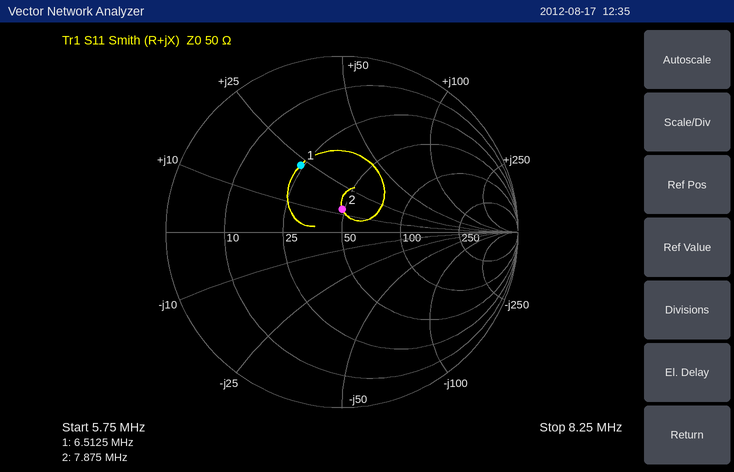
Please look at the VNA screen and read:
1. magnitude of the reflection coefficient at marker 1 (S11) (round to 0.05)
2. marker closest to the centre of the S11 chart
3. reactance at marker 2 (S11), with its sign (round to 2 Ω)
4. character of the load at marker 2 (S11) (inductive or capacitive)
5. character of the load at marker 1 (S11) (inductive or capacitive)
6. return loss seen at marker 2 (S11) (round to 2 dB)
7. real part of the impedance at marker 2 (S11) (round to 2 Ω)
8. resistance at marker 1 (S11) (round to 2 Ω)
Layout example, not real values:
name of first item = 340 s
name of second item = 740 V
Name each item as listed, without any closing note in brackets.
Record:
magnitude of the reflection coefficient at marker 1 (S11) = 0.45
marker closest to the centre of the S11 chart = marker 2
reactance at marker 2 (S11), with its sign = +12 Ω
character of the load at marker 2 (S11) = inductive
character of the load at marker 1 (S11) = inductive
return loss seen at marker 2 (S11) = 18 dB
real part of the impedance at marker 2 (S11) = 48 Ω
resistance at marker 1 (S11) = 24 Ω
